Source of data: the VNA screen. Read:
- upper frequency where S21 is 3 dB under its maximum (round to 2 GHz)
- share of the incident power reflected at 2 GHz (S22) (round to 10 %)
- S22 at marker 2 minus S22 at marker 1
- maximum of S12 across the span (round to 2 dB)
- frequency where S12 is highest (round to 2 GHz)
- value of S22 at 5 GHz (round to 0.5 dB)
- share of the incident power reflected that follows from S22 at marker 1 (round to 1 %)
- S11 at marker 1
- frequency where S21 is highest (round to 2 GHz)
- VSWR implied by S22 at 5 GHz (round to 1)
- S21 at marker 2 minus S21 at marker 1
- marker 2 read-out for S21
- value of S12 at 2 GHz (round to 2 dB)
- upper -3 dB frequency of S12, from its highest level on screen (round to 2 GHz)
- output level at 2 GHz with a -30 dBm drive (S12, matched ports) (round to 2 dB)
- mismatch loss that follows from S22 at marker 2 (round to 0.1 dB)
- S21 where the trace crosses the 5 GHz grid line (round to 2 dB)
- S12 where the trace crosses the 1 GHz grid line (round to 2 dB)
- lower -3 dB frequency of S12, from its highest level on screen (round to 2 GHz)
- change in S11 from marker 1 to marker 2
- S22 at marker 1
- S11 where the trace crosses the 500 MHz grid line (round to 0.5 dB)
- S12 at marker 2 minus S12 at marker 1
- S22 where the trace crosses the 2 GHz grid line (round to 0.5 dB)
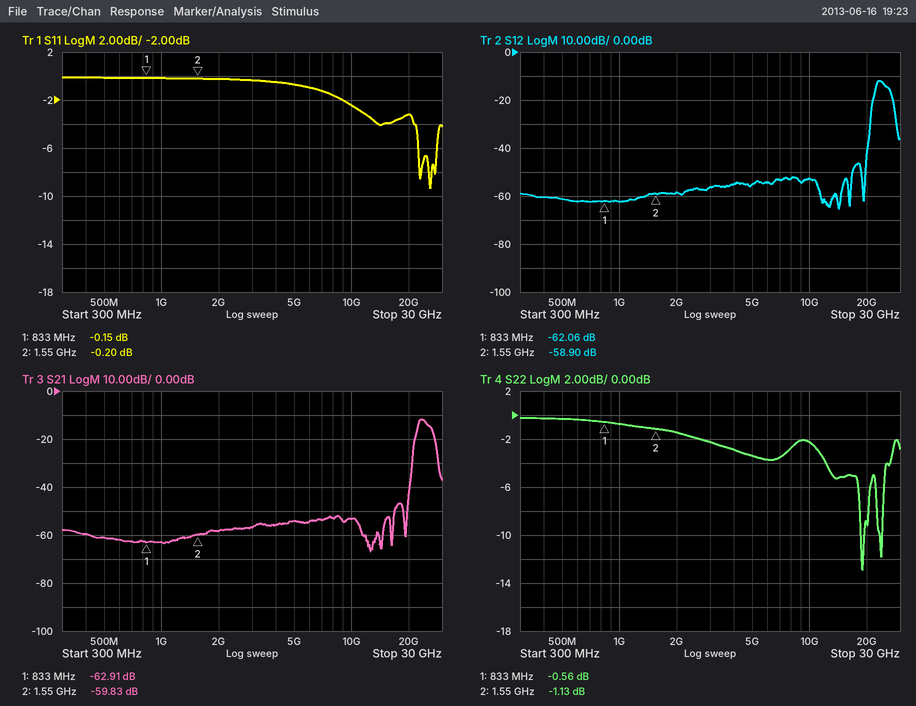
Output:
26 GHz
70 %
-0.57 dB
-12 dB
24 GHz
-3.5 dB
88 %
-0.15 dB
24 GHz
5
3.08 dB
-59.83 dB
-58 dB
26 GHz
-88 dBm
6.4 dB
-54 dB
-62 dB
22 GHz
-0.05 dB
-0.56 dB
0.0 dB
3.16 dB
-1.5 dB
